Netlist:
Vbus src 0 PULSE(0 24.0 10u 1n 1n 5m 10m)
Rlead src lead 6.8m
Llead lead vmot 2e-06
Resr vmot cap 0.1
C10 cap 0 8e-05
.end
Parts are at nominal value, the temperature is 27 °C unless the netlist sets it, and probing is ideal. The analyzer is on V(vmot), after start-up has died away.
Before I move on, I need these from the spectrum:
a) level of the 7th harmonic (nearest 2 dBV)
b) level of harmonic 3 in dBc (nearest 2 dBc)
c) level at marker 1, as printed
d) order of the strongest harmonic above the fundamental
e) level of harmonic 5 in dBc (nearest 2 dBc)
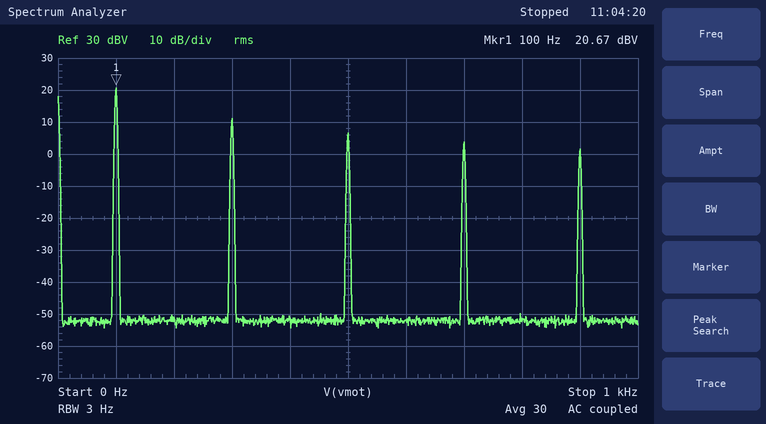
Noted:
4 dBV
-10 dBc
20.67 dBV
3
-14 dBc
